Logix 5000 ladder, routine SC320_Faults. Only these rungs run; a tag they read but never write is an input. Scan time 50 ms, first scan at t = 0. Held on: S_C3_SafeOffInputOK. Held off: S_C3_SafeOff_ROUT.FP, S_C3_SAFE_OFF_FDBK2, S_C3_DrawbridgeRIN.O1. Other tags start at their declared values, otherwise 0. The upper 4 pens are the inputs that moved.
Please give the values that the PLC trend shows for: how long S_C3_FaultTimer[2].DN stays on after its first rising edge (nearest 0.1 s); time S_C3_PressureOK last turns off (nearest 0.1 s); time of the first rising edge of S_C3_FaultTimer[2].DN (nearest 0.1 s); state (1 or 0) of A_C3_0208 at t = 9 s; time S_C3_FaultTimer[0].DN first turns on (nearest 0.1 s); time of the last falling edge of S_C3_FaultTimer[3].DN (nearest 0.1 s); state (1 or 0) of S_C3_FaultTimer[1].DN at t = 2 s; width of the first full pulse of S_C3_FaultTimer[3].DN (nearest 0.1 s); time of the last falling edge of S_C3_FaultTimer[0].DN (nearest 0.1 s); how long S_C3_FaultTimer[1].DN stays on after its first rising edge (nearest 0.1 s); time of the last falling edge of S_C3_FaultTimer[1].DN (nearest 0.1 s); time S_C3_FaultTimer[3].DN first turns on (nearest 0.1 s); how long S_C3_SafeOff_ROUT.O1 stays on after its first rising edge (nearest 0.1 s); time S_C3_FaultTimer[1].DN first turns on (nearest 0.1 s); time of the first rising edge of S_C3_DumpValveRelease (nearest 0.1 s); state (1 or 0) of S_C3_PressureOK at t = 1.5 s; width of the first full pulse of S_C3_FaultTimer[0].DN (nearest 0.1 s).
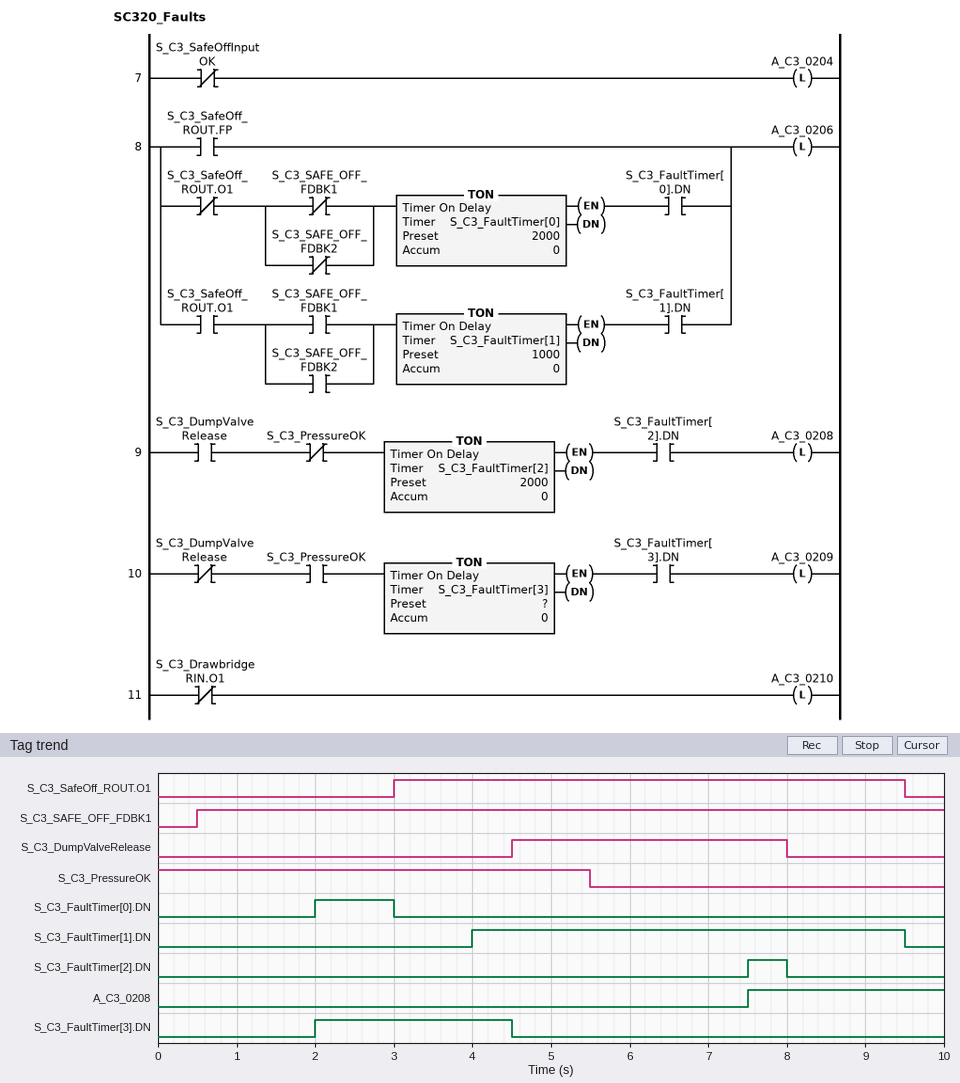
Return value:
0.5 s
5.5 s
7.5 s
1
2.0 s
4.5 s
0
2.5 s
3.0 s
5.5 s
9.5 s
2.0 s
6.5 s
4.0 s
4.5 s
1
1.0 s
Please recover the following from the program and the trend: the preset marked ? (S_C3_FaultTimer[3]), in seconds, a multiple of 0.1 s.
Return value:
2.0 s
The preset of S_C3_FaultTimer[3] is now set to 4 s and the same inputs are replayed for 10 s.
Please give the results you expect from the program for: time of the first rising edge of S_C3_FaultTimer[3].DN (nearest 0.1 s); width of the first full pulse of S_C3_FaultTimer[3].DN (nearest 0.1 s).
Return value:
4.0 s
0.5 s
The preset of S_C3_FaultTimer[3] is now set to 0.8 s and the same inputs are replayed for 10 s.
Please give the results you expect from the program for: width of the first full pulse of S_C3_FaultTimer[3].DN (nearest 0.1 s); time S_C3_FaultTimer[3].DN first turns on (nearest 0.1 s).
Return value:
3.7 s
0.8 s
